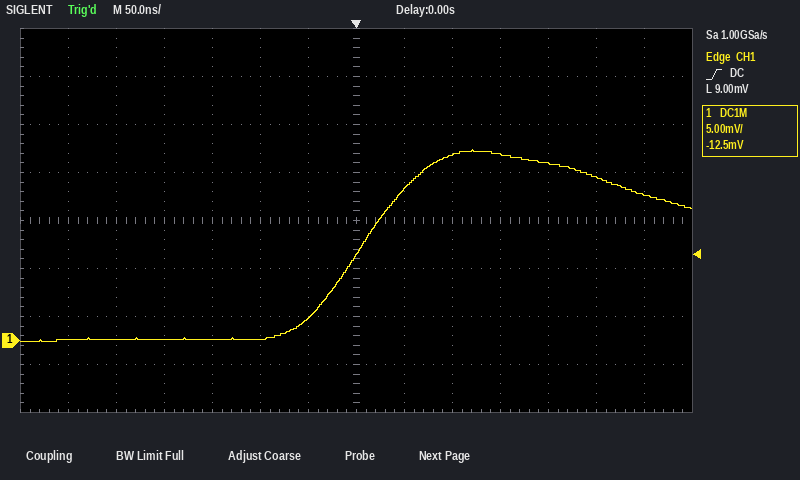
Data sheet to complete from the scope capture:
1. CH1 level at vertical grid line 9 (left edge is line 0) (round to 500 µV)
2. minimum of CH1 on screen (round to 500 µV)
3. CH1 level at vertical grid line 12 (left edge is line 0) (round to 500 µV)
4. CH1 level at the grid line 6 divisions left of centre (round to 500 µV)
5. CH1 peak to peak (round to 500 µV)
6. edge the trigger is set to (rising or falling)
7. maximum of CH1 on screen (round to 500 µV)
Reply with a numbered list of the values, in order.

1. 19.5 mV
2. 0.0 mV
3. 17.0 mV
4. 0.0 mV
5. 20.0 mV
6. rising
7. 20.0 mV
